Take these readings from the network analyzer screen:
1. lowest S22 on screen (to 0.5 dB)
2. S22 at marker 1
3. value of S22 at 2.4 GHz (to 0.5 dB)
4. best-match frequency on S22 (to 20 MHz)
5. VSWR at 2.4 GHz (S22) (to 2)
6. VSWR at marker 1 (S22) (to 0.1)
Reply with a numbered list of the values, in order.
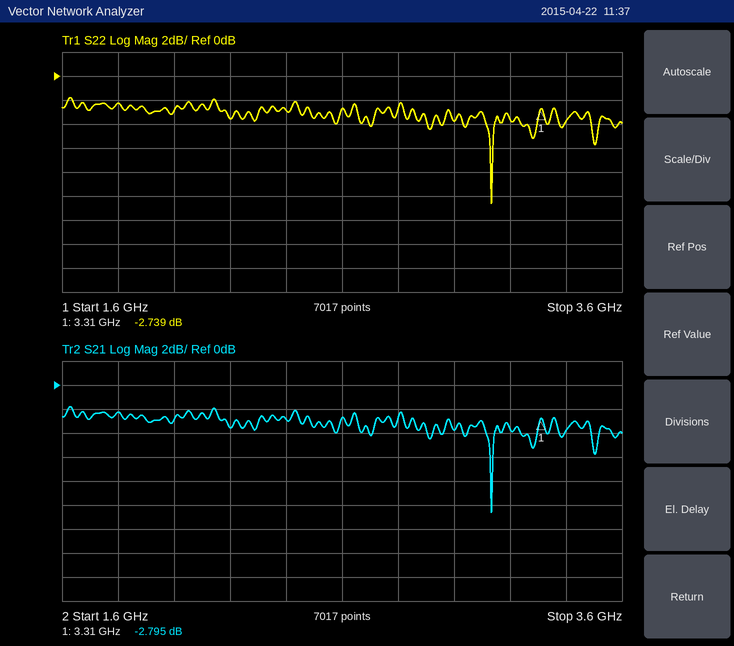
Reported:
1. -10.5 dB
2. -2.739 dB
3. -3.0 dB
4. 3.14 GHz
5. 6
6. 6.4
